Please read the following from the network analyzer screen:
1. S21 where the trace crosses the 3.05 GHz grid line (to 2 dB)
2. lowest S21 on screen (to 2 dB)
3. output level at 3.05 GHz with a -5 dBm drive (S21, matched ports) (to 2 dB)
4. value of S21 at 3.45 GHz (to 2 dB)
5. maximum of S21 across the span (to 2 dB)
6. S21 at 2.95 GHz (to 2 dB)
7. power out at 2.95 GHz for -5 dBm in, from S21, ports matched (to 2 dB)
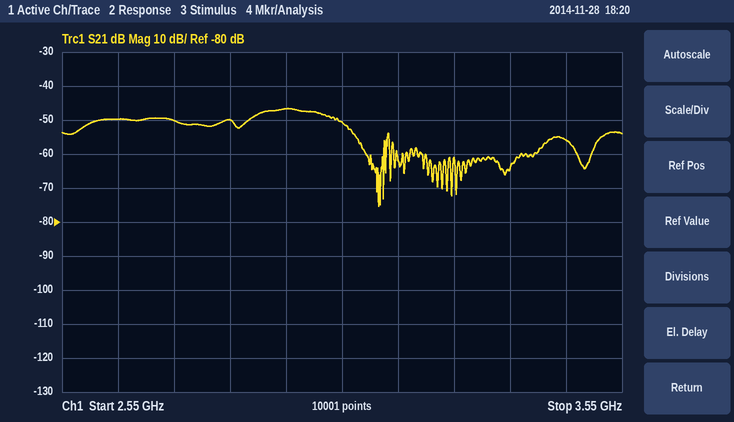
-50 dB
-76 dB
-56 dBm
-56 dB
-46 dB
-46 dB
-52 dBm
